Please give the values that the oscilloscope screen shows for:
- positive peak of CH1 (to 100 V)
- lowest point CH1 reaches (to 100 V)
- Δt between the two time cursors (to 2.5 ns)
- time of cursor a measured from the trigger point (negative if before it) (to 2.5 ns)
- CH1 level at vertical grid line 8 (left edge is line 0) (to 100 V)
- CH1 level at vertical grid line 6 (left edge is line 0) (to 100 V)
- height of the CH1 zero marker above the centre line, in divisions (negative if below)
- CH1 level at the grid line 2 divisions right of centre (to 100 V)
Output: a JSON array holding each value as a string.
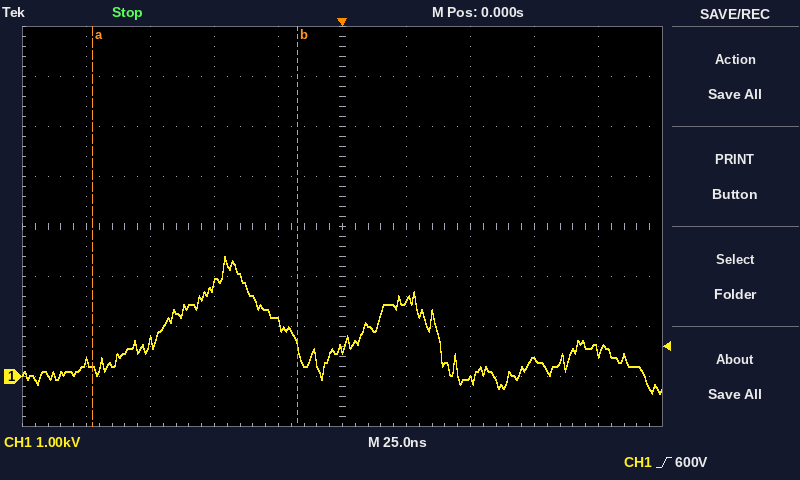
["2.4 kV", "-300 V", "80.0 ns", "-97.5 ns", "300 V", "1.5 kV", "-3.0 div", "-100 V"]
